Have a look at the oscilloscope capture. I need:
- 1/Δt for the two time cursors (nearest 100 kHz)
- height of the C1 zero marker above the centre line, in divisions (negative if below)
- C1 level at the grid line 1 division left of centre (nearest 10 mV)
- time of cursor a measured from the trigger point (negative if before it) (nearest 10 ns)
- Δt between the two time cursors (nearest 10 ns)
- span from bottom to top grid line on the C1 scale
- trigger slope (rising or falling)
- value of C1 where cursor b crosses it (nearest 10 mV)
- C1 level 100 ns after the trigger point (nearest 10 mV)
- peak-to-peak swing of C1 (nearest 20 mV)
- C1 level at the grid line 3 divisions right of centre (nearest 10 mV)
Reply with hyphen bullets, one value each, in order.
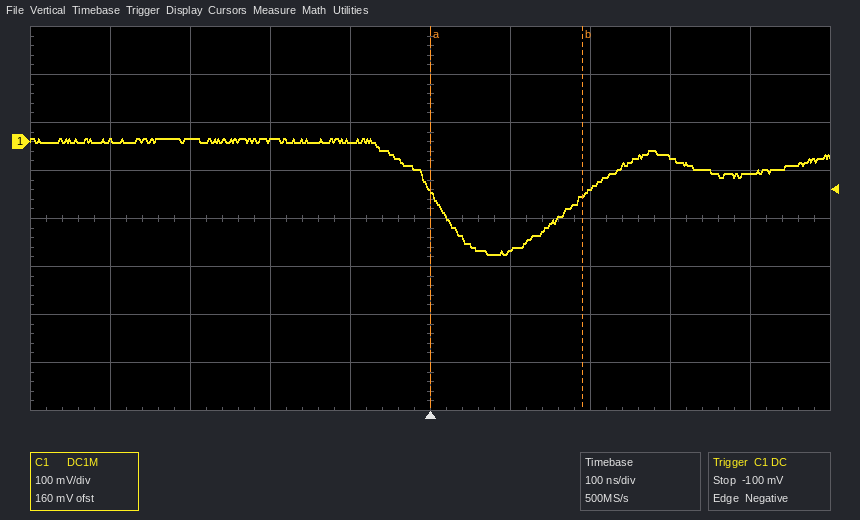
- 5.3 MHz
- +1.6 div
- 0 mV
- 0 ns
- 190 ns
- 800 mV
- falling
- -110 mV
- -230 mV
- 240 mV
- -30 mV
